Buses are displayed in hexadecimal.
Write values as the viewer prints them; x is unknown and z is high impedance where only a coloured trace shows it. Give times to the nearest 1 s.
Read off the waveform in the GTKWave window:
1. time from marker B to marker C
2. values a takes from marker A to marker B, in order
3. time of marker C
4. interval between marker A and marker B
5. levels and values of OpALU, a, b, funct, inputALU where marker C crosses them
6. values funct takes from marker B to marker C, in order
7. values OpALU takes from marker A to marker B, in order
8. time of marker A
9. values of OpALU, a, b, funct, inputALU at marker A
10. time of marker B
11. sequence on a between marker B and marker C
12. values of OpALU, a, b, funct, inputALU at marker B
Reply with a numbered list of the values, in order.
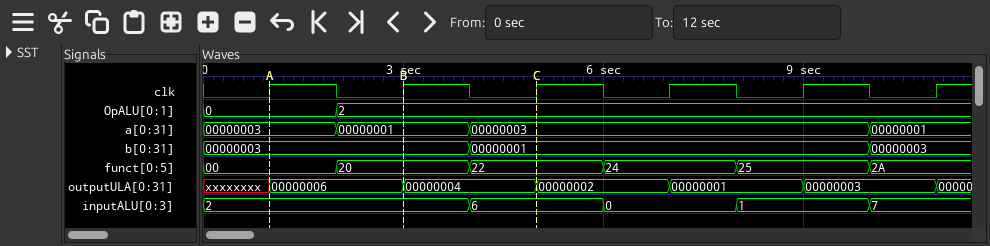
1. 2 s
2. 00000003, 00000001
3. 5 s
4. 2 s
5. OpALU=2, a=00000003, b=00000001, funct=22, inputALU=6
6. 20, 22
7. 0, 2
8. 1 s
9. OpALU=0, a=00000003, b=00000003, funct=00, inputALU=2
10. 3 s
11. 00000001, 00000003
12. OpALU=2, a=00000001, b=00000003, funct=20, inputALU=2
